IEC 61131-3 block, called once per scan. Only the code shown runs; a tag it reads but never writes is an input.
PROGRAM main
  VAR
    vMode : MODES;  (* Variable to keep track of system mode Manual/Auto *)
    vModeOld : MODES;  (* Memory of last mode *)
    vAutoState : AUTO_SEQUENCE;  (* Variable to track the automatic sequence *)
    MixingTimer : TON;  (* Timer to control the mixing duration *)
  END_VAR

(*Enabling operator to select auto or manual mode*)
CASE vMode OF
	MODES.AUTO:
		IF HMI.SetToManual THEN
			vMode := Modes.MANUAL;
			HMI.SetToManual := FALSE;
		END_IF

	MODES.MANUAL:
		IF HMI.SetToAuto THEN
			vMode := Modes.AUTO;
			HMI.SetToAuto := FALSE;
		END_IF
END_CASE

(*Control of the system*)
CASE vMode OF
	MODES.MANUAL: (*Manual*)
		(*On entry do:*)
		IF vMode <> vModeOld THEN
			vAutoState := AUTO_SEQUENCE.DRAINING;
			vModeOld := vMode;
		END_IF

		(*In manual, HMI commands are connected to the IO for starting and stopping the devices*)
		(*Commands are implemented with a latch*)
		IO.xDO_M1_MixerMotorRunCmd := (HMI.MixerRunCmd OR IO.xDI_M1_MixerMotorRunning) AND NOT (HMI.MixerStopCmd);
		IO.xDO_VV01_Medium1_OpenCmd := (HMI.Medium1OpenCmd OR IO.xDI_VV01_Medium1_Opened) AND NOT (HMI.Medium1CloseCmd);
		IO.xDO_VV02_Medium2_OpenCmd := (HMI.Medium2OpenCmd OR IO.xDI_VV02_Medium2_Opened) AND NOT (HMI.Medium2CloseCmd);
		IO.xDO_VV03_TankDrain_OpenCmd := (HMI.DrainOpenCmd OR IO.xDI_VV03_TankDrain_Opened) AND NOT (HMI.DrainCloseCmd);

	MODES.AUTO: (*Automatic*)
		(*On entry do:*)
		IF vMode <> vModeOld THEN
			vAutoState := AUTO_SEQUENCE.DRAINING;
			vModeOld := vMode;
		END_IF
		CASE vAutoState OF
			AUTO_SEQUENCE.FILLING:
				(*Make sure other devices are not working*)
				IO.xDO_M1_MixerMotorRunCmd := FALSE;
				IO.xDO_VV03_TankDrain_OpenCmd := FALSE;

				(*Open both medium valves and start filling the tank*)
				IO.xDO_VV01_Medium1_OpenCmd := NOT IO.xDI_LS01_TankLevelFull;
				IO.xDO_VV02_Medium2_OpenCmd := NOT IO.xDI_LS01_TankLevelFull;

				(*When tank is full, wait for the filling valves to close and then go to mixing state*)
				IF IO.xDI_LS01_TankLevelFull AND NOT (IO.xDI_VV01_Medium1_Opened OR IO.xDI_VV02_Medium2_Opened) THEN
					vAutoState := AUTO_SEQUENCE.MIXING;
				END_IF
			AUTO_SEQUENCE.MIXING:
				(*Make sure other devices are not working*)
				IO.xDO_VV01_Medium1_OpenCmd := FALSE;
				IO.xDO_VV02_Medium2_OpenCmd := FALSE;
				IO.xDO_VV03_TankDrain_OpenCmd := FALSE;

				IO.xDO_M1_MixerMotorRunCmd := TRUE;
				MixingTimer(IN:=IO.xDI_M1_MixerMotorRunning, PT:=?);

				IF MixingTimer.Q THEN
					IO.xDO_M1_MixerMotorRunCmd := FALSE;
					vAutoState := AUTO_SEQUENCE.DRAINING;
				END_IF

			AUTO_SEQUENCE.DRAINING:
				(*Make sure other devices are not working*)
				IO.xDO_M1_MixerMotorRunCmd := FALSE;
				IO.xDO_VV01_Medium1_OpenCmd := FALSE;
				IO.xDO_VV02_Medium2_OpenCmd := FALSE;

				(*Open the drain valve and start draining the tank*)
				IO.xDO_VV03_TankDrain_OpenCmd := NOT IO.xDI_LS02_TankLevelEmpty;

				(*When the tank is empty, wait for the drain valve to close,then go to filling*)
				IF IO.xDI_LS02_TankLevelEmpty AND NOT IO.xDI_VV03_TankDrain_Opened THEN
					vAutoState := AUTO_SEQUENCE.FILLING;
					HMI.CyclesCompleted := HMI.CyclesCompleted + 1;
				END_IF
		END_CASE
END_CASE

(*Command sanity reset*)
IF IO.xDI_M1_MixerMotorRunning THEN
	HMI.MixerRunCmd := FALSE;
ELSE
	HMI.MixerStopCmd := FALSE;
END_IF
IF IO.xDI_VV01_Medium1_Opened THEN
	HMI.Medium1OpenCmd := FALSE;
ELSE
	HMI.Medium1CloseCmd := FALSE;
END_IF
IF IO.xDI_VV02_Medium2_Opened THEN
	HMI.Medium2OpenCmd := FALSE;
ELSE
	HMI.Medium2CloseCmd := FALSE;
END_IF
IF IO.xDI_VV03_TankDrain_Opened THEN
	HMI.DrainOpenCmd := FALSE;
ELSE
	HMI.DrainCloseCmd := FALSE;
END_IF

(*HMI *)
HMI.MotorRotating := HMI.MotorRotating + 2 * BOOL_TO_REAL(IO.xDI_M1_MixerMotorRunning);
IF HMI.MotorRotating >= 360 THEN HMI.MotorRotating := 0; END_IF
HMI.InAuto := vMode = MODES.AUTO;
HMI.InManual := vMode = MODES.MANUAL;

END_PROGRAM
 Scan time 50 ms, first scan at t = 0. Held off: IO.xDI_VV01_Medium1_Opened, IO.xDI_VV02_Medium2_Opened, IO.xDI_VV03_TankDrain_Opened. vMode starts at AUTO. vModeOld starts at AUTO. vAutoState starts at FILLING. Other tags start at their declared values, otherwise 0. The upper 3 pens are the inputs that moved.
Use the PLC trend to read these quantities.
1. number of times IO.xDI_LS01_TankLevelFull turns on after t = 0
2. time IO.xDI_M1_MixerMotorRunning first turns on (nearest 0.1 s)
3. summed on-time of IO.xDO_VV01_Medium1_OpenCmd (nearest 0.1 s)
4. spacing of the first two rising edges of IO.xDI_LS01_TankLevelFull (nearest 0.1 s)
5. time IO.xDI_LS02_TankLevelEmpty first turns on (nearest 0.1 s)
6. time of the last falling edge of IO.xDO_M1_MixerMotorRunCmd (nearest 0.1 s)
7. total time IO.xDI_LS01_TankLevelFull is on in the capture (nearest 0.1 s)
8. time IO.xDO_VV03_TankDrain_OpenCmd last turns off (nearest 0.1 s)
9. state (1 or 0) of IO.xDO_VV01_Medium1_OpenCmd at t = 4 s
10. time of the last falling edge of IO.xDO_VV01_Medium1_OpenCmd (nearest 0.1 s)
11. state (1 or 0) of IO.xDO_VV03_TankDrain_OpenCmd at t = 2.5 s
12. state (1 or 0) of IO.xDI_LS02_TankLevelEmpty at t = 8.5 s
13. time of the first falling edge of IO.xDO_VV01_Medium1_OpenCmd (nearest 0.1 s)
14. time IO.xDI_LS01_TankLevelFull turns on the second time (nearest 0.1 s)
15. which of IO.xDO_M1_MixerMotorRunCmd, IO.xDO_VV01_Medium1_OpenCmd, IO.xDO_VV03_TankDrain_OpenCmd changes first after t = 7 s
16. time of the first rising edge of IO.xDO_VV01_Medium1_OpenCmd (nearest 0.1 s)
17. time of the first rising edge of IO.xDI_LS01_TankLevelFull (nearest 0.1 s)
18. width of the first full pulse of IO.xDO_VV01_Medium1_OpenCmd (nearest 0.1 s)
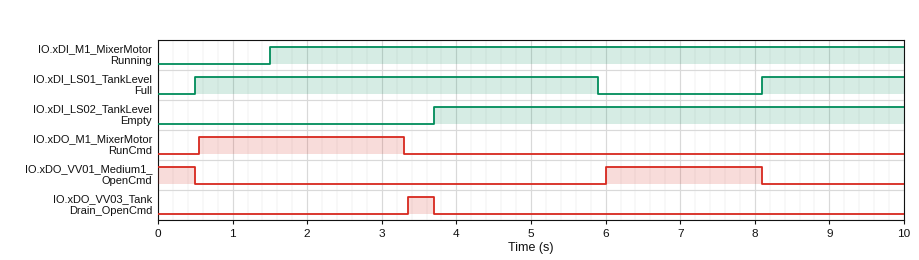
2
1.5 s
2.6 s
7.6 s
3.7 s
3.3 s
7.3 s
3.7 s
0
8.1 s
0
1
0.5 s
8.1 s
IO.xDO_VV01_Medium1_OpenCmd
6.0 s
0.5 s
2.1 s
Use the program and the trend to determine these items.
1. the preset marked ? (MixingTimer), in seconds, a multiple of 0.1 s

1.8 s
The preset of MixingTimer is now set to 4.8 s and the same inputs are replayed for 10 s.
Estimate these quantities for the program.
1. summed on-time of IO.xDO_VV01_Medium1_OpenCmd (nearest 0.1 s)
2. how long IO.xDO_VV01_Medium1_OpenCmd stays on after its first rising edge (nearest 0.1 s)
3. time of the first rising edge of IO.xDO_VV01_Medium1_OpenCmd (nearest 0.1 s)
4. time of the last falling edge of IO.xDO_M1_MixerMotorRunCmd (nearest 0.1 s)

2.2 s
1.7 s
6.4 s
6.3 s
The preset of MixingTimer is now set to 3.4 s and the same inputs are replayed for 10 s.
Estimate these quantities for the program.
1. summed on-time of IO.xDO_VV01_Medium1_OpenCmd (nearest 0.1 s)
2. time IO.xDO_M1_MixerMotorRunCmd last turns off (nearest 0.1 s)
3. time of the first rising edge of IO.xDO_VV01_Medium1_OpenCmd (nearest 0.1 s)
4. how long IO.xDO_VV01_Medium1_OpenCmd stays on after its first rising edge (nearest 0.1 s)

2.7 s
4.9 s
5.9 s
2.2 s
